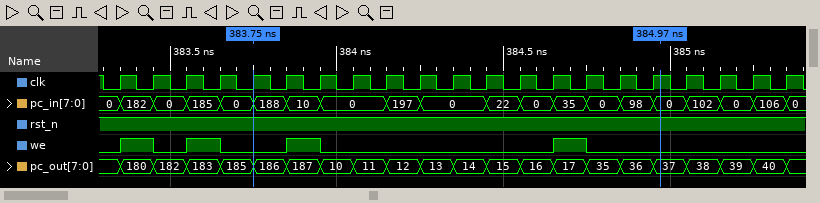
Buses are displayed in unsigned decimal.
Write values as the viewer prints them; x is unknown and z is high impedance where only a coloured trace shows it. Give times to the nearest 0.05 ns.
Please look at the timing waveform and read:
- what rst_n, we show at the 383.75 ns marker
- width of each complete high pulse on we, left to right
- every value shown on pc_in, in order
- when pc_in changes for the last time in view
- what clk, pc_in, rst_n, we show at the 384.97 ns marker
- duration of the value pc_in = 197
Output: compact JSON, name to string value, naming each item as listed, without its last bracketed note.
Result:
{"what rst_n, we show at the 383.75 ns marker": "rst_n=1, we=0", "width of each complete high pulse on we, left to right": "0.1 ns, 0.1 ns, 0.1 ns, 0.1 ns", "every value shown on pc_in, in order": "0, 182, 0, 185, 0, 188, 10, 0, 197, 0, 22, 0, 35, 0, 98, 0, 102, 0, 106, 0", "when pc_in changes for the last time in view": "385.35 ns", "what clk, pc_in, rst_n, we show at the 384.97 ns marker": "clk=1, pc_in=0, rst_n=1, we=0", "duration of the value pc_in = 197": "0.1 ns"}
